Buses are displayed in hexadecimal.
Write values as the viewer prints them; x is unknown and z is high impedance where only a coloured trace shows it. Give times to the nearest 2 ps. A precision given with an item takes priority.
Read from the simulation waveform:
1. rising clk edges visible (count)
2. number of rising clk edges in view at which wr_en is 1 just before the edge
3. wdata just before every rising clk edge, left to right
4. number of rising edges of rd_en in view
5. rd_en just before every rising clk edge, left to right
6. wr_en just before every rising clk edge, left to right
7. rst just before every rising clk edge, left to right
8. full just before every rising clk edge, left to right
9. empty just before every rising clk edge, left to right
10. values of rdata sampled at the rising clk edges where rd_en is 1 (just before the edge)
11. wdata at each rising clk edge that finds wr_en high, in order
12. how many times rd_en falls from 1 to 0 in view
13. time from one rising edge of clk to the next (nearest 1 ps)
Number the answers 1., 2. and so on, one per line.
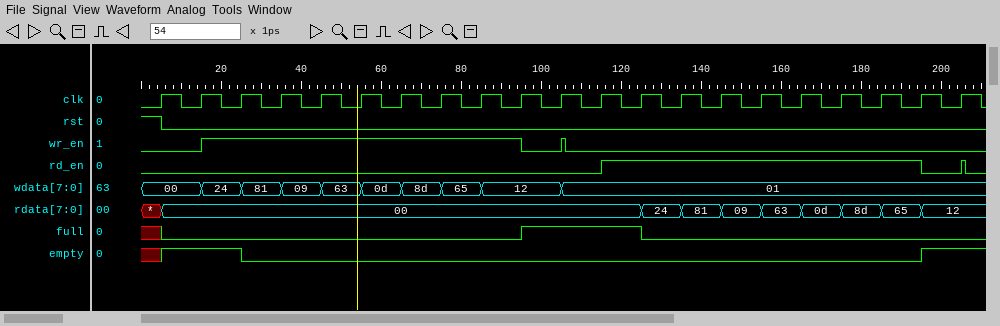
1. 21
2. 8
3. 00, 00, 24, 81, 09, 63, 0d, 8d, 65, 12, 12, 01, 01, 01, 01, 01, 01, 01, 01, 01, 01
4. 2
5. 0 0 0 0 0 0 0 0 0 0 0 0 1 1 1 1 1 1 1 1 0
6. 0 0 1 1 1 1 1 1 1 1 0 0 0 0 0 0 0 0 0 0 0
7. 1 0 0 0 0 0 0 0 0 0 0 0 0 0 0 0 0 0 0 0 0
8. x 0 0 0 0 0 0 0 0 0 1 1 1 0 0 0 0 0 0 0 0
9. x 1 1 0 0 0 0 0 0 0 0 0 0 0 0 0 0 0 0 0 1
10. 00, 24, 81, 09, 63, 0d, 8d, 65
11. 24, 81, 09, 63, 0d, 8d, 65, 12
12. 2
13. 10 ps
